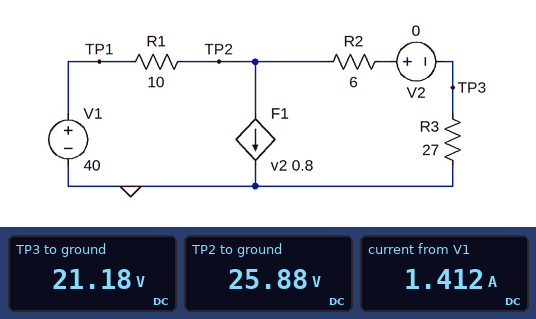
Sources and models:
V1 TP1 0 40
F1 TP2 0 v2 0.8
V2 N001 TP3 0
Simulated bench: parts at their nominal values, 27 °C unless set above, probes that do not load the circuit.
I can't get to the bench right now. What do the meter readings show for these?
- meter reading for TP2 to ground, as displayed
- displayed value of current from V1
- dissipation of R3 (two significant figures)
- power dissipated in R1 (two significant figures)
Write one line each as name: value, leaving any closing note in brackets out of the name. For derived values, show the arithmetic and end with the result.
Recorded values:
meter reading for TP2 to ground, as displayed: 25.88 V
displayed value of current from V1: 1.412 A
dissipation of R3: (21.18 V)^2 / 27 Ω = 17 W
power dissipated in R1: (40 V - 25.88 V)^2 / 10 Ω = 20 W
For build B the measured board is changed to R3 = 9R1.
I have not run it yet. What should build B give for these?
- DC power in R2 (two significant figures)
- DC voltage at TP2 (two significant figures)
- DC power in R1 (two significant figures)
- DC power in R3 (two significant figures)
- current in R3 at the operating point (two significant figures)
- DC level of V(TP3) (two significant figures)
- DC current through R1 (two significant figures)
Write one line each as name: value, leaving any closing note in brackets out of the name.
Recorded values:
DC power in R2: 8.8 W
DC voltage at TP2: 18 V
DC power in R1: 47 W
DC power in R3: 13 W
current in R3 at the operating point: 1.2 A
DC level of V(TP3): 11 V
DC current through R1: 2.2 A
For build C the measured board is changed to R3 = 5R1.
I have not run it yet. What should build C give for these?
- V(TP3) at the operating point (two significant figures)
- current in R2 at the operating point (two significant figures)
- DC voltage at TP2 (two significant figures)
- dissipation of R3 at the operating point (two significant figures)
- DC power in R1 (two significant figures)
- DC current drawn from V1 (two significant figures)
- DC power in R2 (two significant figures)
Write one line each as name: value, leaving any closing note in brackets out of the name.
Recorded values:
V(TP3) at the operating point: 7.0 V
current in R2 at the operating point: 1.4 A
DC voltage at TP2: 15 V
dissipation of R3 at the operating point: 9.6 W
DC power in R1: 61 W
DC current drawn from V1: 2.5 A
DC power in R2: 11 W
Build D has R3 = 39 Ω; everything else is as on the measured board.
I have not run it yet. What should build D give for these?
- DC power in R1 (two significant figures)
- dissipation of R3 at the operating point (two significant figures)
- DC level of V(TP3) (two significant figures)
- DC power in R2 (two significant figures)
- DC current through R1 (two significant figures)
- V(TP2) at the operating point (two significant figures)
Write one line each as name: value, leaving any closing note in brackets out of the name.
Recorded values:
DC power in R1: 13 W
dissipation of R3 at the operating point: 16 W
DC level of V(TP3): 25 V
DC power in R2: 2.4 W
DC current through R1: 1.1 A
V(TP2) at the operating point: 29 V
